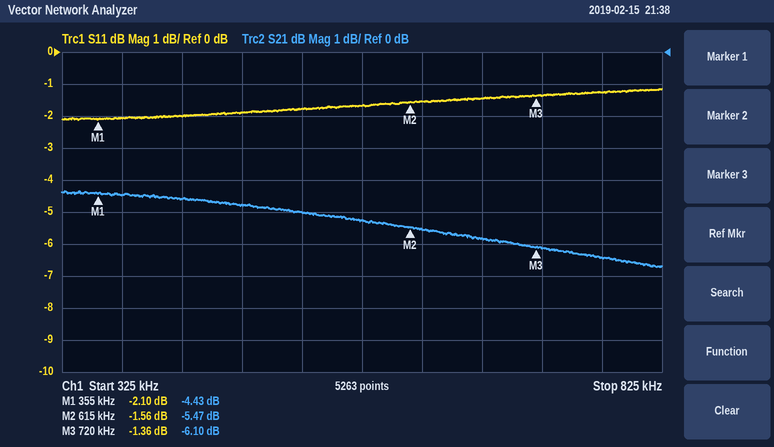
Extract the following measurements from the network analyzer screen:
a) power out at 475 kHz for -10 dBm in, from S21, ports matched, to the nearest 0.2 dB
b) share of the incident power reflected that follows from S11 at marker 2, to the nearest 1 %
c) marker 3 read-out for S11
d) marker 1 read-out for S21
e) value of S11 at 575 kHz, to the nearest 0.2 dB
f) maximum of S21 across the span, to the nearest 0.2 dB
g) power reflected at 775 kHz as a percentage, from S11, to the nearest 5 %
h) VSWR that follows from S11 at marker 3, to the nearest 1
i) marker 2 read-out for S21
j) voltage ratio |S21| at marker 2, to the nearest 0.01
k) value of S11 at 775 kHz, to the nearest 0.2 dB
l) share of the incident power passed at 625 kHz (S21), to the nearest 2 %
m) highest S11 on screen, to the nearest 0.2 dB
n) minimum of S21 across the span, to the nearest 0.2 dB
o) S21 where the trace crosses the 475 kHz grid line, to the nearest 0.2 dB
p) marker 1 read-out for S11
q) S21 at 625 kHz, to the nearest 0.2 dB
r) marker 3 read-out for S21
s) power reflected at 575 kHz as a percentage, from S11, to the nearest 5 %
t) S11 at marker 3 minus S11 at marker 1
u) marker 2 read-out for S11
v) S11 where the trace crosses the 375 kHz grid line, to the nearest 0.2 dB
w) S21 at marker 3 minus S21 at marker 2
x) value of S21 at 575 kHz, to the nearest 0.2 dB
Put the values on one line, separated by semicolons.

-14.8 dBm; 70 %; -1.36 dB; -4.43 dB; -1.6 dB; -4.4 dB; 75 %; 13; -5.47 dB; 0.53; -1.2 dB; 28 %; -1.2 dB; -6.8 dB; -4.8 dB; -2.10 dB; -5.6 dB; -6.10 dB; 70 %; 0.74 dB; -1.56 dB; -2.0 dB; -0.63 dB; -5.2 dB
